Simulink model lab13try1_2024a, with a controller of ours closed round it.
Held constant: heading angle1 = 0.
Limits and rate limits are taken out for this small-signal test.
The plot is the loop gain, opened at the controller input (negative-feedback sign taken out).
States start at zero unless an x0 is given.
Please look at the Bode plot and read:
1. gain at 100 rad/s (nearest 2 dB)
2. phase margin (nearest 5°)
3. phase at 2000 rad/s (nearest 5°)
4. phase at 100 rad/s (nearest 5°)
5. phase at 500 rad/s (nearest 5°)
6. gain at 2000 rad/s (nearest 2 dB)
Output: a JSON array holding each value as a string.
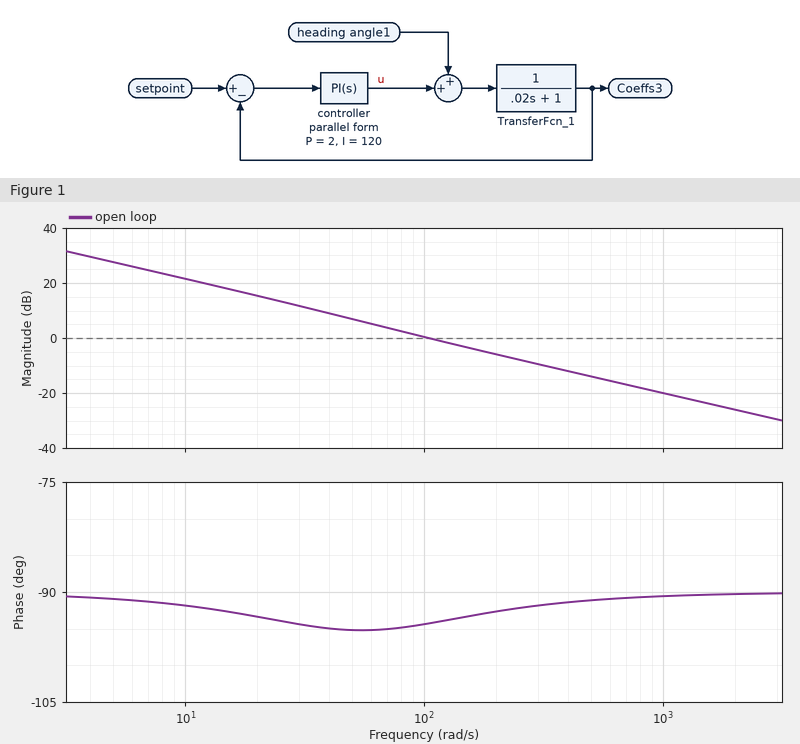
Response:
["0 dB", "85°", "-90°", "-95°", "-90°", "-26 dB"]
